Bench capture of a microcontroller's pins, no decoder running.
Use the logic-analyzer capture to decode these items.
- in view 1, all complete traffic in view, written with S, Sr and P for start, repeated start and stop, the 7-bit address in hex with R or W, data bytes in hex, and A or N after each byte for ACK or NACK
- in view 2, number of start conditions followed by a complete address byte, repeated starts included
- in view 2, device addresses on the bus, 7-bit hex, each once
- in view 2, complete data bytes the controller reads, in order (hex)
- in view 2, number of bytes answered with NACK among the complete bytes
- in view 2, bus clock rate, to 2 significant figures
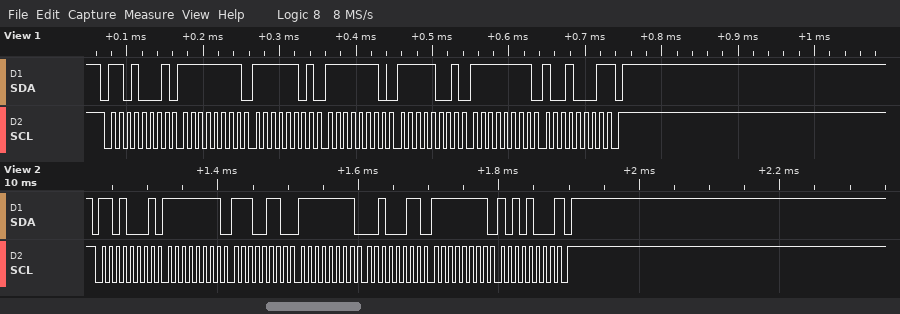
S 68R A FF A FD A FE A F9 A FF A 91 N P
1
0x68
FF E6 FF 23 FF A8
1
100 kHz
